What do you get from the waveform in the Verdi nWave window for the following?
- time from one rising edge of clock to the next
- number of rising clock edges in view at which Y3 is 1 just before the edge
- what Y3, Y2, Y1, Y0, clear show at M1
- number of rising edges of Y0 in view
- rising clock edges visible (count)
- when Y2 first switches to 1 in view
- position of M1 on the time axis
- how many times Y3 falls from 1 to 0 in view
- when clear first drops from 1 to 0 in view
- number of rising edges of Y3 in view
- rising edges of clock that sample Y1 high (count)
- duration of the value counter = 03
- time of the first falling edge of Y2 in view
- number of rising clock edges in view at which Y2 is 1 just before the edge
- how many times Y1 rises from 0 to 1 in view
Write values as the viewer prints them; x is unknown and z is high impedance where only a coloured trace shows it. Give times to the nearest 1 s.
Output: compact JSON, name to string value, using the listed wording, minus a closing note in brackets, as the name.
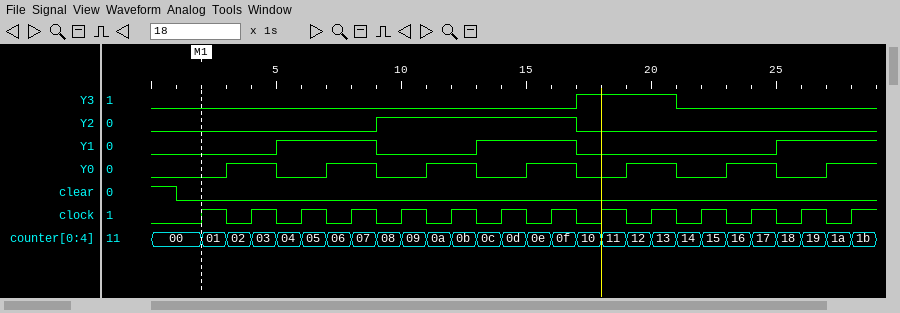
{"time from one rising edge of clock to the next": "2 s", "number of rising clock edges in view at which Y3 is 1 just before the edge": "2", "what Y3, Y2, Y1, Y0, clear show at M1": "Y3=0, Y2=0, Y1=0, Y0=0, clear=0", "number of rising edges of Y0 in view": "7", "rising clock edges visible": "14", "when Y2 first switches to 1 in view": "9 s", "position of M1 on the time axis": "2 s", "how many times Y3 falls from 1 to 0 in view": "1", "when clear first drops from 1 to 0 in view": "1 s", "number of rising edges of Y3 in view": "1", "rising edges of clock that sample Y1 high": "6", "duration of the value counter = 03": "1 s", "time of the first falling edge of Y2 in view": "17 s", "number of rising clock edges in view at which Y2 is 1 just before the edge": "4", "how many times Y1 rises from 0 to 1 in view": "3"}
